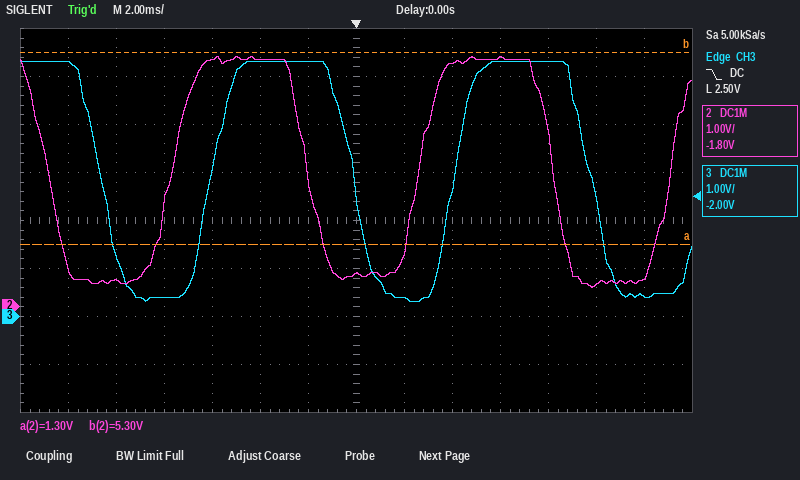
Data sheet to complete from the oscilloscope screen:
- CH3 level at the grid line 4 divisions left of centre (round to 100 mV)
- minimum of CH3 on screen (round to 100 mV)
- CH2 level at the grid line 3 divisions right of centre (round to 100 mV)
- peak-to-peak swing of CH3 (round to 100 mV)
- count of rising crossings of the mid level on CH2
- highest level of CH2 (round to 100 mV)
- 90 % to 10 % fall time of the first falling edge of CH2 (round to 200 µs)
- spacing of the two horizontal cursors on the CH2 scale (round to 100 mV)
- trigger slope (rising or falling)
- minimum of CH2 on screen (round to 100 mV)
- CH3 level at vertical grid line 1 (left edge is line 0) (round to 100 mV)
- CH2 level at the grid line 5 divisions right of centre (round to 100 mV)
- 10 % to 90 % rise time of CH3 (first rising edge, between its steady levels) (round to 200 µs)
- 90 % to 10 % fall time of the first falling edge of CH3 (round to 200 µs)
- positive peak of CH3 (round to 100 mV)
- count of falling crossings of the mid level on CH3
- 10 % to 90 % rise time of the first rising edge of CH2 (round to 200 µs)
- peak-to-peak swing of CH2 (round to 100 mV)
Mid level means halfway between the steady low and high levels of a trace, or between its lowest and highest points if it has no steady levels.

400 mV
300 mV
5.2 V
5.0 V
3
5.2 V
1.6 ms
4.0 V
falling
400 mV
5.3 V
500 mV
1.6 ms
1.8 ms
5.3 V
3
1.8 ms
4.8 V
